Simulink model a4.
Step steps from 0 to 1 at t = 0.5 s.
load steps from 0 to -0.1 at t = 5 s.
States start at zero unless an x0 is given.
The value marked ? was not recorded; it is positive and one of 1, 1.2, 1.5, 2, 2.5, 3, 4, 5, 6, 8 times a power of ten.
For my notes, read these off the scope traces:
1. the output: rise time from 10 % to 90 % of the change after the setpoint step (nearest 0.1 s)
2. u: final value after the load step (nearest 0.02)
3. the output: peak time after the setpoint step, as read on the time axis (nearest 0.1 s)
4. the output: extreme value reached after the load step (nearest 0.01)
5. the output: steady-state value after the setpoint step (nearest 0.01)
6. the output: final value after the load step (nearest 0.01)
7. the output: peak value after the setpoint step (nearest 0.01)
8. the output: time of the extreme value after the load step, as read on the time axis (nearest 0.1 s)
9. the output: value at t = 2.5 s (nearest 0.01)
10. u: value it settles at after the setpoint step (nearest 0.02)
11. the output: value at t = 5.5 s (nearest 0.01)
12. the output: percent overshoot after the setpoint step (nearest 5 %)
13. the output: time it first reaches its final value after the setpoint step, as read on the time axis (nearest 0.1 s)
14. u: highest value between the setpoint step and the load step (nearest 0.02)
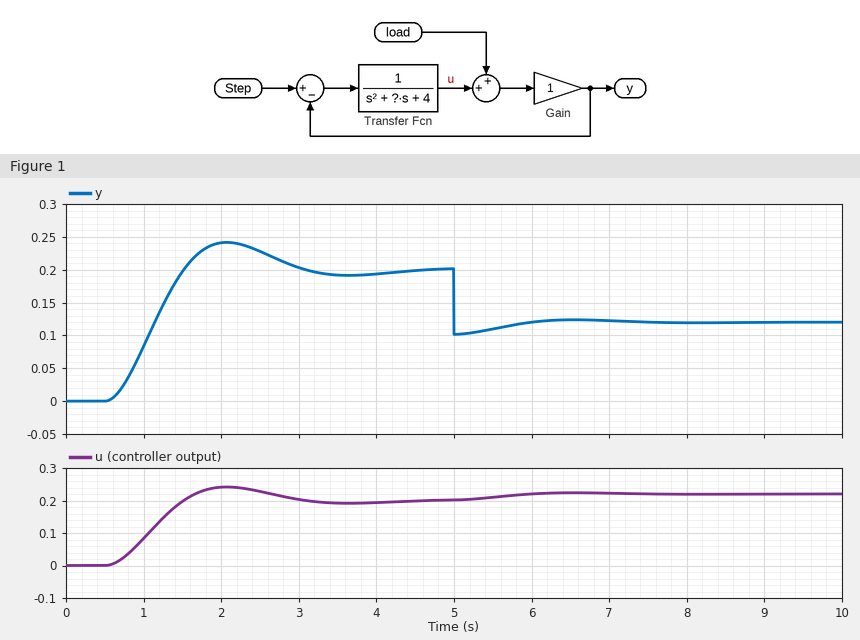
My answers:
0.7 s
0.22
2.1 s
0.10
0.20
0.12
0.24
5.0 s
0.23
0.20
0.11
20 %
1.5 s
0.24
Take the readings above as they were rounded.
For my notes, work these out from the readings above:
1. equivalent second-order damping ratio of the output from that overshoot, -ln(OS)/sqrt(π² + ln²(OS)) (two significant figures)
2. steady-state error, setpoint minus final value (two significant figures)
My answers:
0.46
0.80
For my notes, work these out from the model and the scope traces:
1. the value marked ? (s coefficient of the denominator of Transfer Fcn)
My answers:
2
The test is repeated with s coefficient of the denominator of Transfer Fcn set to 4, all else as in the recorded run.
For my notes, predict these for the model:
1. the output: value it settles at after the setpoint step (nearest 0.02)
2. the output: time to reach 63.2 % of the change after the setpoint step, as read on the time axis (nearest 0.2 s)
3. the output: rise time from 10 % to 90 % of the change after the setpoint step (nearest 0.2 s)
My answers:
0.20
1.4 s
1.2 s
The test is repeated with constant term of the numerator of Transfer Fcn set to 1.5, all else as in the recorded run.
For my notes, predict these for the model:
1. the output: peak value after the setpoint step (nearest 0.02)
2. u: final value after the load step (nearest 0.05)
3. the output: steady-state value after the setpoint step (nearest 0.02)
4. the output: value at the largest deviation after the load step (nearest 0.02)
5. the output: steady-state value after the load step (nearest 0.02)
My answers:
0.34
0.30
0.28
0.18
0.20
